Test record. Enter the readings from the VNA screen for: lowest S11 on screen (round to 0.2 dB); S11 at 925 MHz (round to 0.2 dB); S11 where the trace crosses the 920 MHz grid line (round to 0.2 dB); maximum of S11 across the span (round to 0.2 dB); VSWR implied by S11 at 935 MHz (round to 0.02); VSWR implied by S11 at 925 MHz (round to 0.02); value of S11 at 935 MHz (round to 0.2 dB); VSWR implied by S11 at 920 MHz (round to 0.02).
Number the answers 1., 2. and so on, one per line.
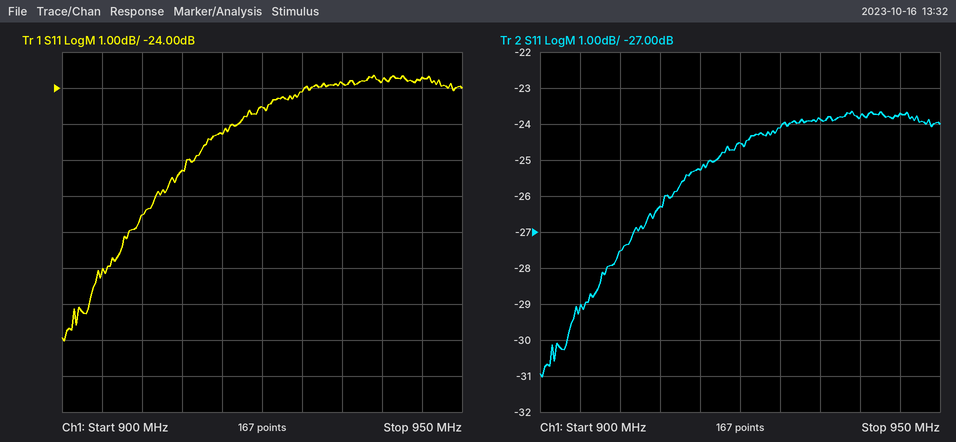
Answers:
1. -31.0 dB
2. -24.6 dB
3. -25.2 dB
4. -23.6 dB
5. 1.14
6. 1.12
7. -23.8 dB
8. 1.12
